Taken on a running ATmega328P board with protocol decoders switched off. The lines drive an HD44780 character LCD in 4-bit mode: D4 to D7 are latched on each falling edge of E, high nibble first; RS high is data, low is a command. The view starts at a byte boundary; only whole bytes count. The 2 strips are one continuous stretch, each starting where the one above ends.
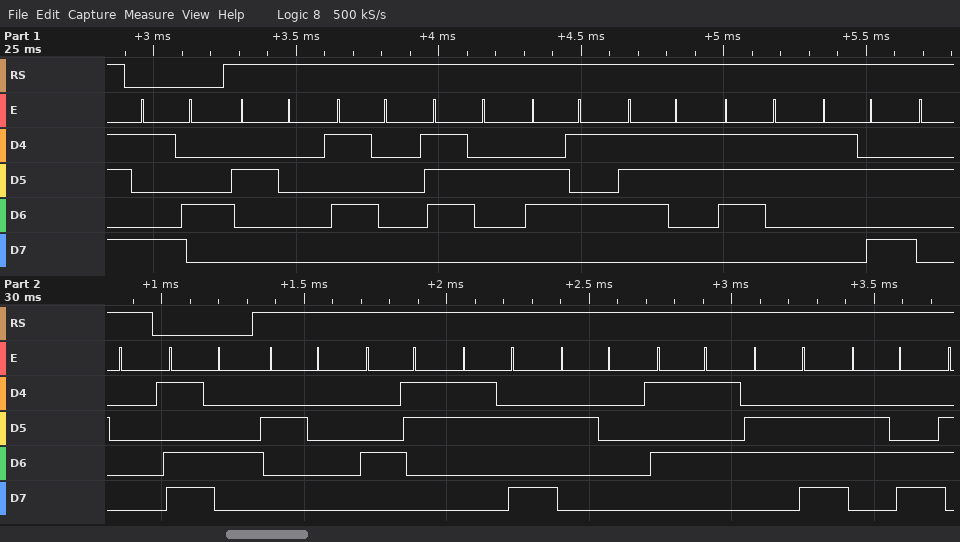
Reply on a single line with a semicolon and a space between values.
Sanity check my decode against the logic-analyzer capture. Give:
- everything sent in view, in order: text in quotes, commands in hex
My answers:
0x94 " Press: " 0xD4 " C: Unl"
